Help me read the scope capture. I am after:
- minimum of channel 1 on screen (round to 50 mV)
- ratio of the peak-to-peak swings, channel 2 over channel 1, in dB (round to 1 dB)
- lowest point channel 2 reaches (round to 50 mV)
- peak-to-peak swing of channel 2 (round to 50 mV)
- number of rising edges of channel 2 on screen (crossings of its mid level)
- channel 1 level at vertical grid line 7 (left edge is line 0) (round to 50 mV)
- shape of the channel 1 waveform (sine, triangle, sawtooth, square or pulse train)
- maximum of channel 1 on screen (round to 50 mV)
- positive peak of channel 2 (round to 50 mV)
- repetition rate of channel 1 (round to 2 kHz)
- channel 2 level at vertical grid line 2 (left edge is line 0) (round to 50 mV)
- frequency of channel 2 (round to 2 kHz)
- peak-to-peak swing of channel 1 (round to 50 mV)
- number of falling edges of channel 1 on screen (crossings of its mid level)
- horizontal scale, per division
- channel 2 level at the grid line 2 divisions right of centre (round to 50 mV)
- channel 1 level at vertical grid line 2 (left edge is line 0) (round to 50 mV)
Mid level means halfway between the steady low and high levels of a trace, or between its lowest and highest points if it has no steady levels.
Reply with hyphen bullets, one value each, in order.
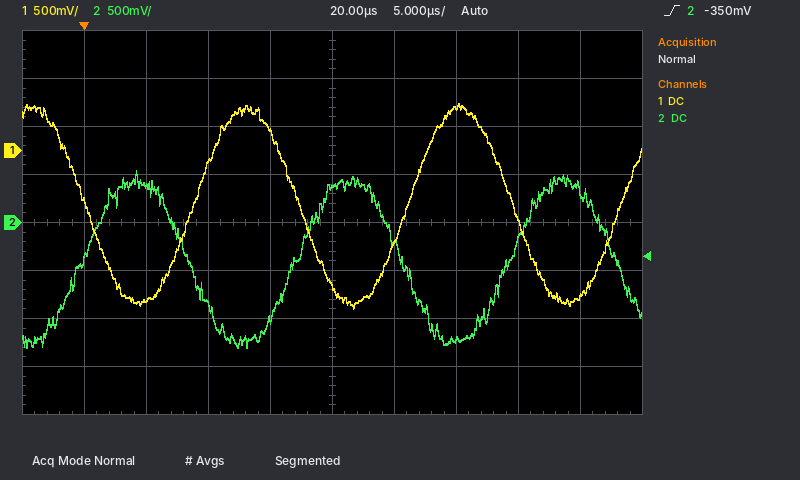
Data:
- -1.65 V
- -1 dB
- -1.30 V
- 1.85 V
- 3
- 450 mV
- sine
- 500 mV
- 550 mV
- 58 kHz
- 400 mV
- 58 kHz
- 2.15 V
- 3
- 5 µs
- -1.20 V
- -1.55 V
